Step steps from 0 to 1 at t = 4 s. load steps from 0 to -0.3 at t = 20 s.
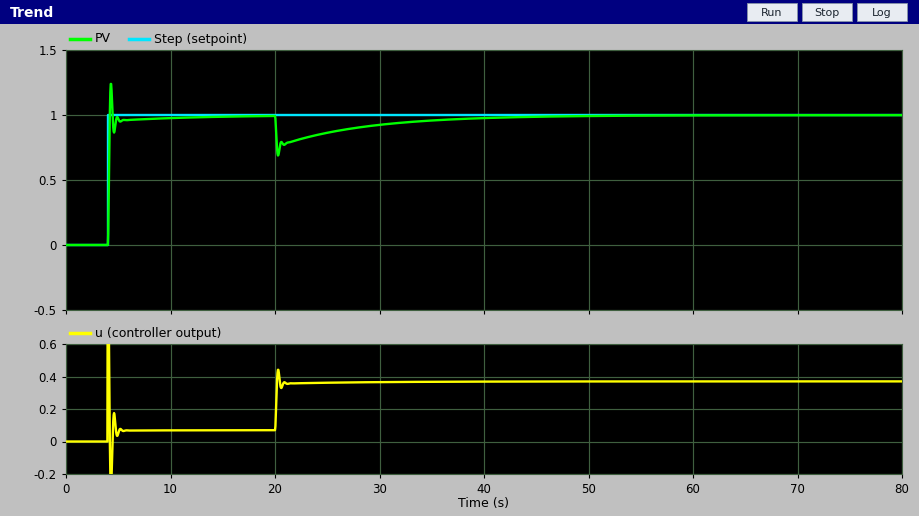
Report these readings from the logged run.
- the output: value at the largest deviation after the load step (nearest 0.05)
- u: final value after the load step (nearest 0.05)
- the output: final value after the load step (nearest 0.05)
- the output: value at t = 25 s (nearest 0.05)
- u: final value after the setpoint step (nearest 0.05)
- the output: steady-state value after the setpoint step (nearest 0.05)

0.70
0.35
1.00
0.85
0.05
1.00
